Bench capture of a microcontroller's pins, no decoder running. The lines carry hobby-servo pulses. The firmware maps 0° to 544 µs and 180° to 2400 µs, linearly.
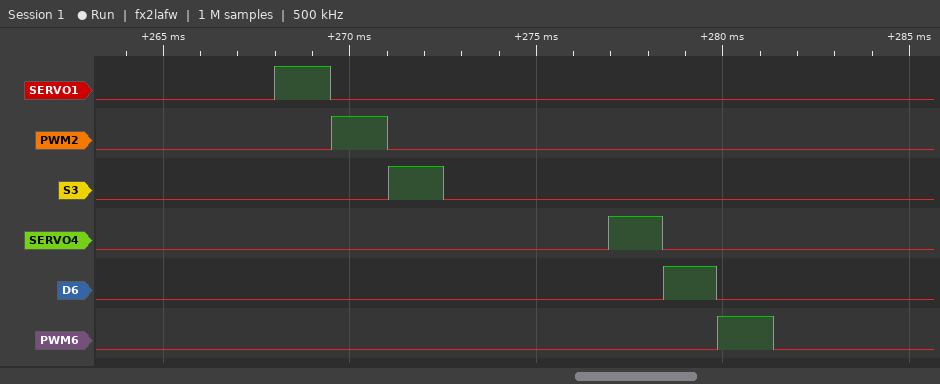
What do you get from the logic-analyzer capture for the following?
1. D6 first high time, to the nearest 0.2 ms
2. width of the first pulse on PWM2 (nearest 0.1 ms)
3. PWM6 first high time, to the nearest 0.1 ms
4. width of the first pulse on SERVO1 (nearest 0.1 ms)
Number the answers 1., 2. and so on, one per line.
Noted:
1. 1.4 ms
2. 1.5 ms
3. 1.5 ms
4. 1.5 ms
